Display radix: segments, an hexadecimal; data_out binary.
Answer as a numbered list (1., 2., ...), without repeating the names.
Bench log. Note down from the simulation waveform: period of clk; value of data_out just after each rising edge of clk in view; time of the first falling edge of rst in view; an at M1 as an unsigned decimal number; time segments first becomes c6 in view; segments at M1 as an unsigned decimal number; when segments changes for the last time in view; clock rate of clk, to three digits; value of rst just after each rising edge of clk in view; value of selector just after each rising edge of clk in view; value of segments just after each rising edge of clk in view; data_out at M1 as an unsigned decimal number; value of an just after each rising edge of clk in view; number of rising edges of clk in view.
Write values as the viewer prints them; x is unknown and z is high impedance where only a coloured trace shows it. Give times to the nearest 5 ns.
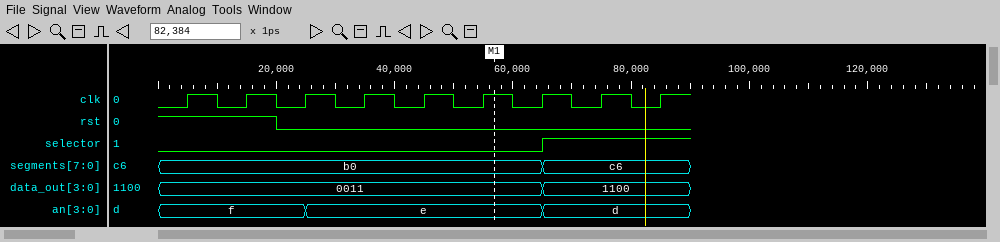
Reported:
1. 10 ns
2. 0011, 0011, 0011, 0011, 0011, 0011, 1100, 1100, 1100
3. 20 ns
4. 14
5. 65 ns
6. 176
7. 65 ns
8. 100 MHz
9. 1 1 0 0 0 0 0 0 0
10. 0 0 0 0 0 0 1 1 1
11. b0, b0, b0, b0, b0, b0, c6, c6, c6
12. 3
13. f, f, e, e, e, e, d, d, d
14. 9
